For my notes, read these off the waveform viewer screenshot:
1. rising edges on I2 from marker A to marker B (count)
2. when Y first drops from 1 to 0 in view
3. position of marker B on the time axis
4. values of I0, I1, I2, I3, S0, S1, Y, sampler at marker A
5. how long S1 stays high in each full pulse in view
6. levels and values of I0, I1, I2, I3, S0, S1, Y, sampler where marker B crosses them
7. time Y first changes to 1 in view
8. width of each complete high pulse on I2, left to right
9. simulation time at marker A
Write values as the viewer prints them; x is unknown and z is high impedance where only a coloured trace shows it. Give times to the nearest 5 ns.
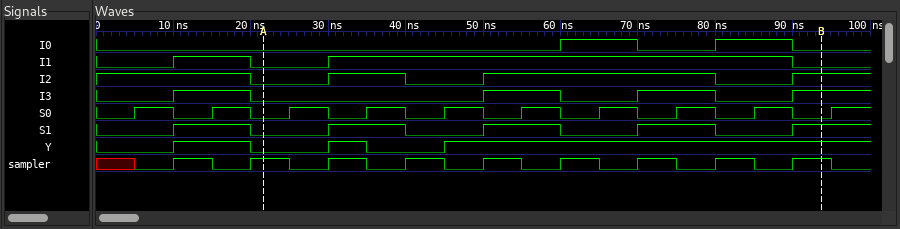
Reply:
3
20 ns
95 ns
I0=0, I1=0, I2=0, I3=0, S0=0, S1=0, Y=0, sampler=1
10 ns, 10 ns, 10 ns, 10 ns
I0=0, I1=0, I2=1, I3=1, S0=0, S1=1, Y=1, sampler=1
10 ns
10 ns, 30 ns
20 ns
